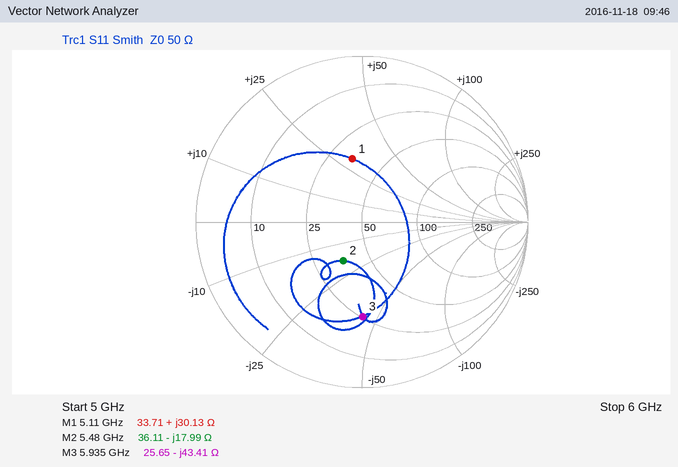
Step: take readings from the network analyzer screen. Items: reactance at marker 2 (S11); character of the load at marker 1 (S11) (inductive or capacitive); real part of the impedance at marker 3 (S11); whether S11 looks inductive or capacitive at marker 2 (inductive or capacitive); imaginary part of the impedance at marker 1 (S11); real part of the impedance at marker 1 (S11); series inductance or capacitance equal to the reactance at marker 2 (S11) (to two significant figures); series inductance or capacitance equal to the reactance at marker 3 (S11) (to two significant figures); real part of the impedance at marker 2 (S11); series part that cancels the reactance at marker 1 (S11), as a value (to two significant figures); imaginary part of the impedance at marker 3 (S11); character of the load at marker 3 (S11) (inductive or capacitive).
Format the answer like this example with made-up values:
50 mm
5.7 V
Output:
-17.99 Ω
inductive
25.65 Ω
capacitive
+30.13 Ω
33.71 Ω
1.6 pF
620 fF
36.11 Ω
1.0 pF
-43.41 Ω
capacitive
